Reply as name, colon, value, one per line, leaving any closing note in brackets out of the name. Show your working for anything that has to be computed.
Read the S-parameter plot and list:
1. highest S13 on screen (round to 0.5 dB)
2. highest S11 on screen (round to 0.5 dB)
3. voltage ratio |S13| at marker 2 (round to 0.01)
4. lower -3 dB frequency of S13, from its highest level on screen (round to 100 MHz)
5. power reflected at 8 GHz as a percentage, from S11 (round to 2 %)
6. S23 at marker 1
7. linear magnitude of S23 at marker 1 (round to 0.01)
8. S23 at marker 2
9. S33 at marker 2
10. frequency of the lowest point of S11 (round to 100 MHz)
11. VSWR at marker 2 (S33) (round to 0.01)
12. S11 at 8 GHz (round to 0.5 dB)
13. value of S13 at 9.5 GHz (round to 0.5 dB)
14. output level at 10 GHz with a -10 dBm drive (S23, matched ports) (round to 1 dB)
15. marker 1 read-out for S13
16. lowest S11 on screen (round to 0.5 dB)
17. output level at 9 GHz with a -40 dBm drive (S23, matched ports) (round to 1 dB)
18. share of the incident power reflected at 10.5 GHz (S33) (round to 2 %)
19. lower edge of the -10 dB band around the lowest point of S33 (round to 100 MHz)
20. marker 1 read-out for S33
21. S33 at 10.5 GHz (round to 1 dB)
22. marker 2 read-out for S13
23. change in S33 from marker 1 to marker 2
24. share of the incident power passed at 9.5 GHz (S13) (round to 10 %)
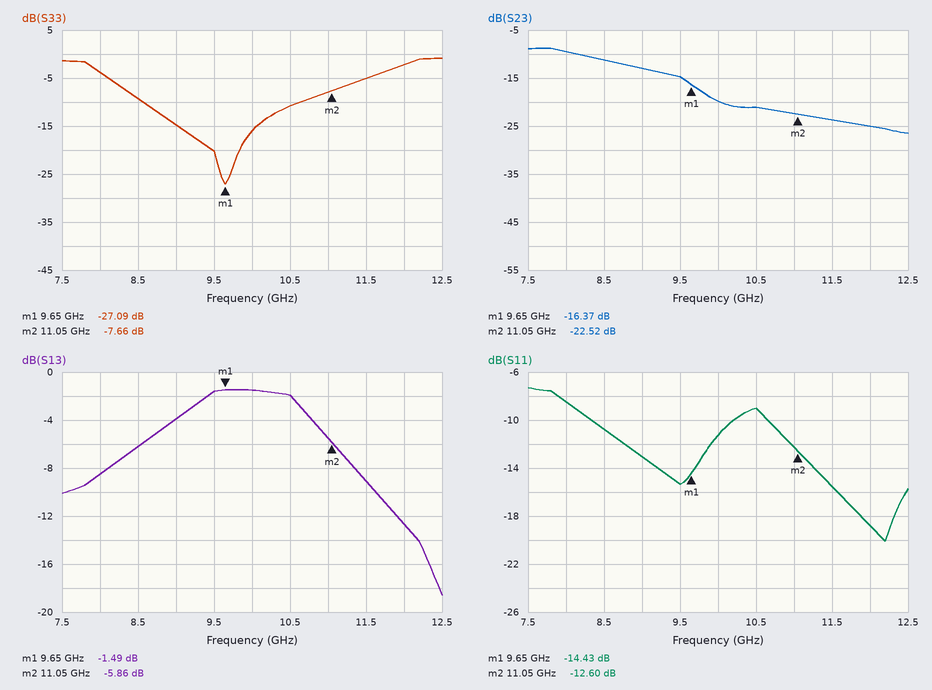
highest S13 on screen: -1.5 dB
highest S11 on screen: -7.5 dB
voltage ratio |S13| at marker 2: 10^(-5.86/20) ≈ 0.51
lower -3 dB frequency of S13, from its highest level on screen: 8.9 GHz
power reflected at 8 GHz as a percentage, from S11: 10^(-8.5/10) ≈ 14 %
S23 at marker 1: -16.37 dB
linear magnitude of S23 at marker 1: 10^(-16.37/20) ≈ 0.15
S23 at marker 2: -22.52 dB
S33 at marker 2: -7.66 dB
frequency of the lowest point of S11: 12.2 GHz
VSWR at marker 2 (S33): (1 + 0.4140)/(1 − 0.4140) ≈ 2.41
S11 at 8 GHz: -8.5 dB
value of S13 at 9.5 GHz: -1.5 dB
output level at 10 GHz with a -10 dBm drive (S23, matched ports): -10 dBm + (-20 dB) = -30 dBm
marker 1 read-out for S13: -1.49 dB
lowest S11 on screen: -20.0 dB
output level at 9 GHz with a -40 dBm drive (S23, matched ports): -40 dBm + (-13 dB) = -53 dBm
share of the incident power reflected at 10.5 GHz (S33): 10^(-11/10) ≈ 8 %
lower edge of the -10 dB band around the lowest point of S33: 8.6 GHz
marker 1 read-out for S33: -27.09 dB
S33 at 10.5 GHz: -11 dB
marker 2 read-out for S13: -5.86 dB
change in S33 from marker 1 to marker 2: -7.66 − (-27.09) = 19.43 dB
share of the incident power passed at 9.5 GHz (S13): 10^(-1.5/10) ≈ 70.8 %, so 70 % to the nearest 10 %
